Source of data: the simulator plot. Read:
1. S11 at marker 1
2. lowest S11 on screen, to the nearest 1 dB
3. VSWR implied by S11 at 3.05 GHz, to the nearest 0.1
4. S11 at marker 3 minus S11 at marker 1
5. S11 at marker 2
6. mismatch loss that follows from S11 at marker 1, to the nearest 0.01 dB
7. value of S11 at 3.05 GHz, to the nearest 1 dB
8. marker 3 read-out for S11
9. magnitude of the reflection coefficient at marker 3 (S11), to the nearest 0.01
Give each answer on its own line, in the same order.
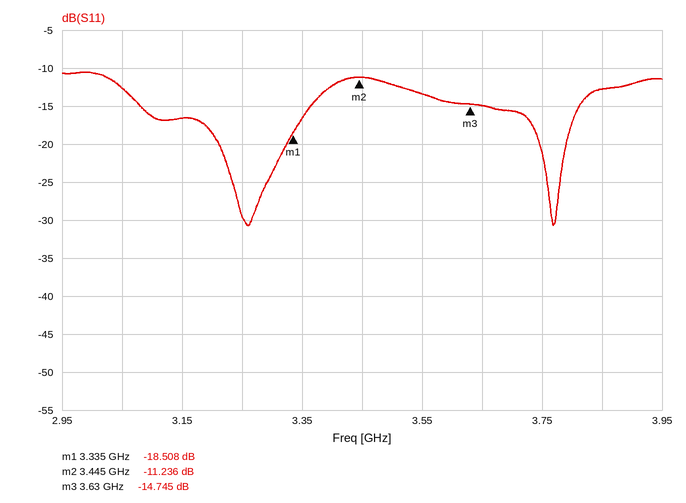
-18.508 dB
-31 dB
1.6
3.763 dB
-11.236 dB
0.06 dB
-13 dB
-14.745 dB
0.18
